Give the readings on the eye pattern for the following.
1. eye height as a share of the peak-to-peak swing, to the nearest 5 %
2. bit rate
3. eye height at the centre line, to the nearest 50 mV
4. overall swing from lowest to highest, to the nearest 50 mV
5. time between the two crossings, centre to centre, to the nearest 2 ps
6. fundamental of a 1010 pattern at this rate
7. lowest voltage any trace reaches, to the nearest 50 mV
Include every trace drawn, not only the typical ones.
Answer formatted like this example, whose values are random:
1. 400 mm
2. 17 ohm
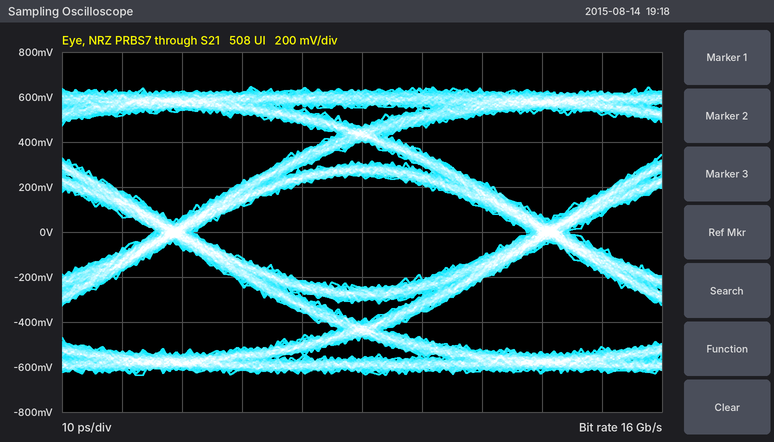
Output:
1. 40 %
2. 16 Gb/s
3. 500 mV
4. 1.30 V
5. 62 ps
6. 8 GHz
7. -650 mV
